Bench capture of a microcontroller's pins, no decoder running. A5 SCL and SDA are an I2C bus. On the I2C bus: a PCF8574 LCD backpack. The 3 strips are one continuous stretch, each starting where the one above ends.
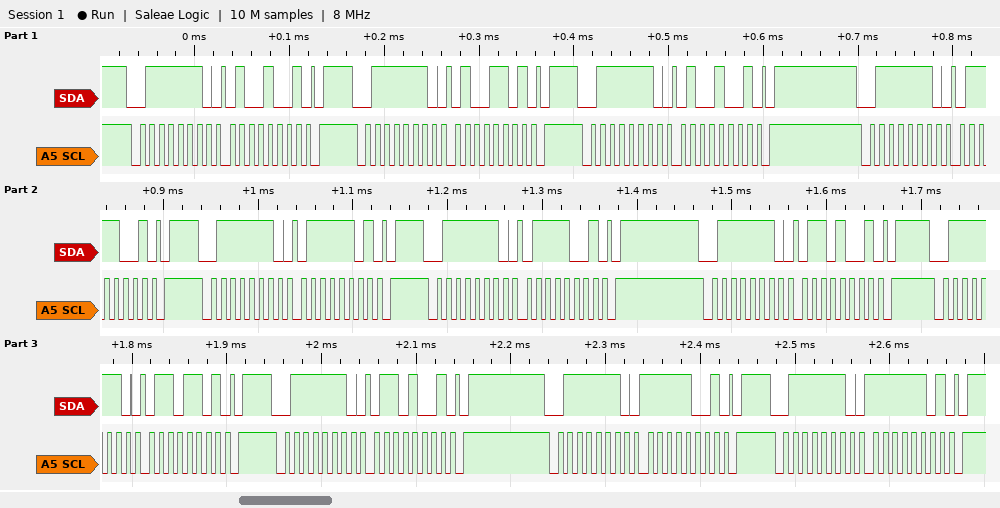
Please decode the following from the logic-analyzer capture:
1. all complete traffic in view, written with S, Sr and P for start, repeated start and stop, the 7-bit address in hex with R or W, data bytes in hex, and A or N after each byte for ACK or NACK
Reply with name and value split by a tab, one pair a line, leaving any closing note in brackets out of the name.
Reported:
all complete traffic in view, written with S, Sr and P for start, repeated start and stop, the 7-bit address in hex with R or W, data bytes in hex, and A or N after each byte for ACK or NACK	S 3FW A 49 A P S 3FW A 4D A P S 3FW A 49 A P S 3FW A 79 A P S 3FW A 7D A P S 3FW A 79 A P S 3FW A 69 A P S 3FW A 6D A P S 3FW A 69 A P S 3FW A F9 A P S 3FW A FD A P
